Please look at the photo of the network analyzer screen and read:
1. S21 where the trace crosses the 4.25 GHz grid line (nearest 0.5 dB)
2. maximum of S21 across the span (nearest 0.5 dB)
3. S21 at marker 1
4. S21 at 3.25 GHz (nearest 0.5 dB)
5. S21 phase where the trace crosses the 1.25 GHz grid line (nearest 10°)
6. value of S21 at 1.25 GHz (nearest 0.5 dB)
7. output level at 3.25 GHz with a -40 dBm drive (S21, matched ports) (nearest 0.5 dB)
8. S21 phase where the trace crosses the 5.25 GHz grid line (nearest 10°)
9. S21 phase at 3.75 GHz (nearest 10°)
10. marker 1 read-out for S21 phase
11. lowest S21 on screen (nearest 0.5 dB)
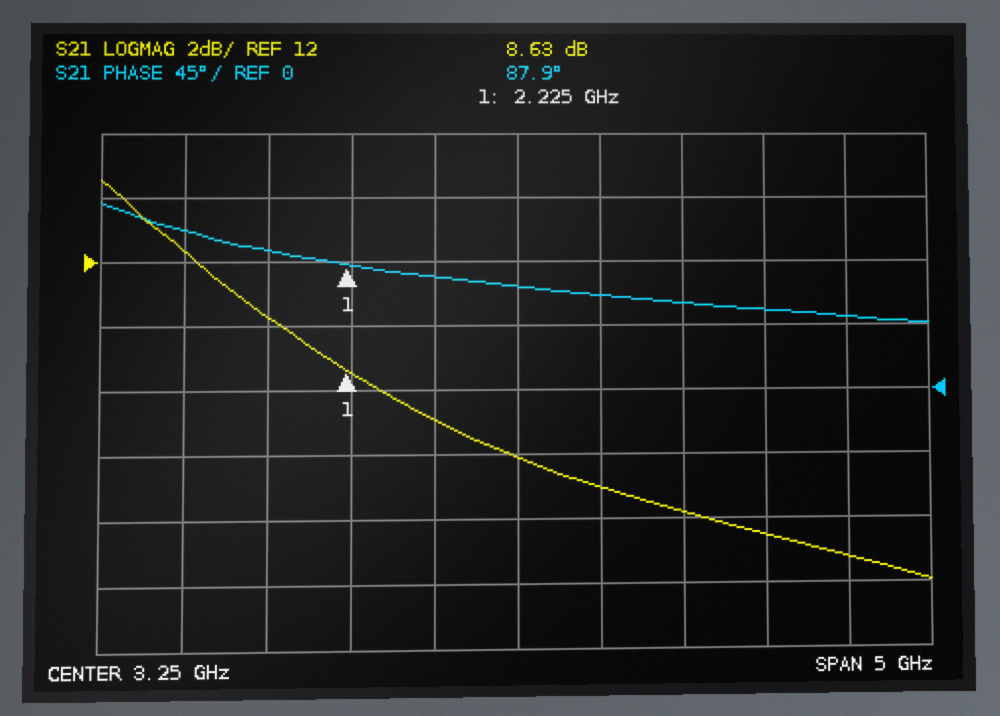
4.0 dB
14.5 dB
8.63 dB
6.0 dB
110°
12.5 dB
-34.0 dBm
50°
70°
87.9°
2.0 dB
